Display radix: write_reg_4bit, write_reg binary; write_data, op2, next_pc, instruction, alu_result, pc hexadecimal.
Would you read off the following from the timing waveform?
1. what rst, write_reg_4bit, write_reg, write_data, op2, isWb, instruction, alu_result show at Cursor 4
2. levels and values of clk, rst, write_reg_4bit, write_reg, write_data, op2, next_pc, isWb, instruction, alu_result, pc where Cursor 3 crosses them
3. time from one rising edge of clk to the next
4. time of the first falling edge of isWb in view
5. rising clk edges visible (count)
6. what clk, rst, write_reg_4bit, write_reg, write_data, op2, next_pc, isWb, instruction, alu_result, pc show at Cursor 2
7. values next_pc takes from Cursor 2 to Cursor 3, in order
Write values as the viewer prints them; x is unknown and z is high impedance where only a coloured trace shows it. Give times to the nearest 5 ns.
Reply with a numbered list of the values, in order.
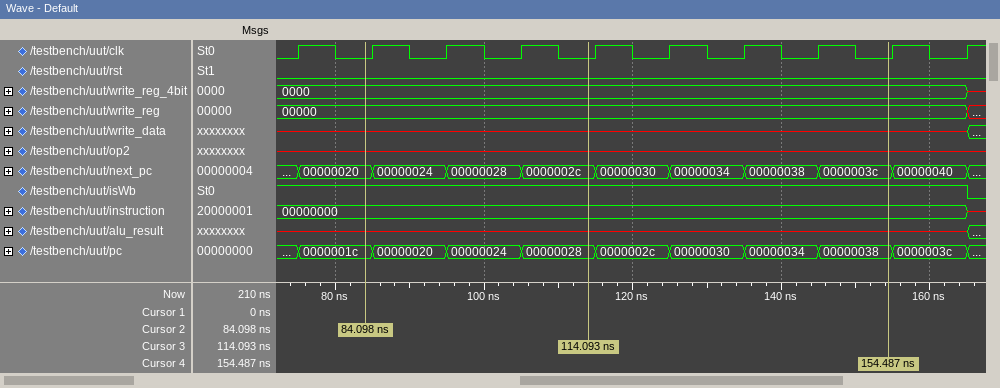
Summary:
1. rst=0, write_reg_4bit=0000, write_reg=00000, write_data=x, op2=x, isWb=1, instruction=00000000, alu_result=x
2. clk=0, rst=0, write_reg_4bit=0000, write_reg=00000, write_data=x, op2=x, next_pc=0000002c, isWb=1, instruction=00000000, alu_result=x, pc=00000028
3. 10 ns
4. 165 ns
5. 10
6. clk=0, rst=0, write_reg_4bit=0000, write_reg=00000, write_data=x, op2=x, next_pc=00000020, isWb=1, instruction=00000000, alu_result=x, pc=0000001c
7. 00000020, 00000024, 00000028, 0000002c
